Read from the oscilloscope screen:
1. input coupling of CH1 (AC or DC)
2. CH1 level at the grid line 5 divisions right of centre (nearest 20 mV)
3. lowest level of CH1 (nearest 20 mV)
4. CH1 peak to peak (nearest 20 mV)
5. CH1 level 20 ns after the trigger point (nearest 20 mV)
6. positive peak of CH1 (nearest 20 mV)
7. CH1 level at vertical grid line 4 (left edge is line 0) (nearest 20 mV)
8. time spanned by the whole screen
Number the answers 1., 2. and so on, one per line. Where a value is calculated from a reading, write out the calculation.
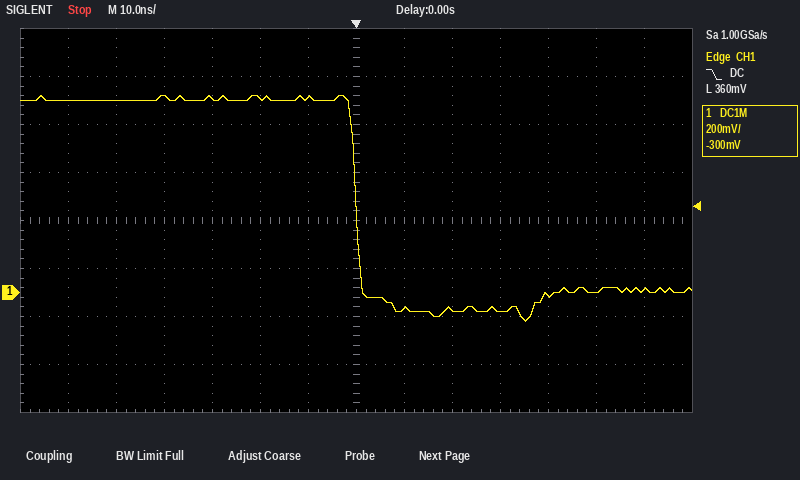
1. DC
2. 0 mV
3. -120 mV
4. 820 mV − (-120 mV) = 940 mV
5. -80 mV
6. 820 mV
7. 800 mV
8. 140 ns
